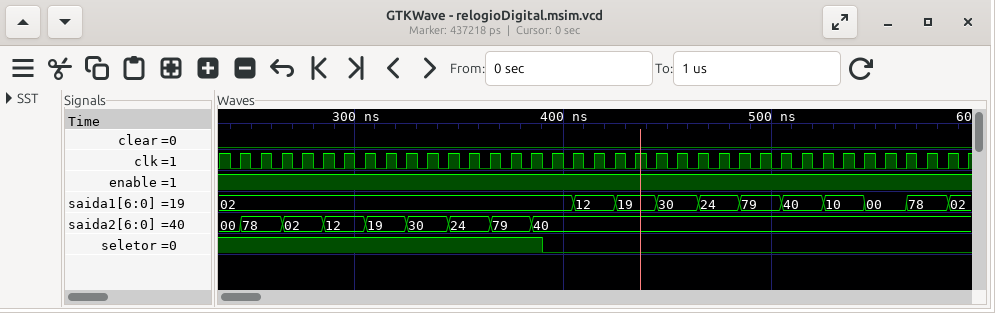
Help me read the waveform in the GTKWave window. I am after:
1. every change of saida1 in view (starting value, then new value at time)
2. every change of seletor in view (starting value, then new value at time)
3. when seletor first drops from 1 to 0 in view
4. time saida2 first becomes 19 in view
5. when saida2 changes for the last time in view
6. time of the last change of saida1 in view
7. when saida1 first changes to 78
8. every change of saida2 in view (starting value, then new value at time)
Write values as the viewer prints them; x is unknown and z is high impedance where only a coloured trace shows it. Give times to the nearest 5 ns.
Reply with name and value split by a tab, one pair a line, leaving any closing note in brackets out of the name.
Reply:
every change of saida1 in view	02, 12 at 405 ns, 19 at 425 ns, 30 at 445 ns, 24 at 465 ns, 79 at 485 ns, 40 at 505 ns, 10 at 525 ns, 00 at 545 ns, 78 at 565 ns, 02 at 585 ns
every change of seletor in view	1, 0 at 390 ns
when seletor first drops from 1 to 0 in view	390 ns
time saida2 first becomes 19 in view	305 ns
when saida2 changes for the last time in view	385 ns
time of the last change of saida1 in view	585 ns
when saida1 first changes to 78	565 ns
every change of saida2 in view	00, 78 at 245 ns, 02 at 265 ns, 12 at 285 ns, 19 at 305 ns, 30 at 325 ns, 24 at 345 ns, 79 at 365 ns, 40 at 385 ns
